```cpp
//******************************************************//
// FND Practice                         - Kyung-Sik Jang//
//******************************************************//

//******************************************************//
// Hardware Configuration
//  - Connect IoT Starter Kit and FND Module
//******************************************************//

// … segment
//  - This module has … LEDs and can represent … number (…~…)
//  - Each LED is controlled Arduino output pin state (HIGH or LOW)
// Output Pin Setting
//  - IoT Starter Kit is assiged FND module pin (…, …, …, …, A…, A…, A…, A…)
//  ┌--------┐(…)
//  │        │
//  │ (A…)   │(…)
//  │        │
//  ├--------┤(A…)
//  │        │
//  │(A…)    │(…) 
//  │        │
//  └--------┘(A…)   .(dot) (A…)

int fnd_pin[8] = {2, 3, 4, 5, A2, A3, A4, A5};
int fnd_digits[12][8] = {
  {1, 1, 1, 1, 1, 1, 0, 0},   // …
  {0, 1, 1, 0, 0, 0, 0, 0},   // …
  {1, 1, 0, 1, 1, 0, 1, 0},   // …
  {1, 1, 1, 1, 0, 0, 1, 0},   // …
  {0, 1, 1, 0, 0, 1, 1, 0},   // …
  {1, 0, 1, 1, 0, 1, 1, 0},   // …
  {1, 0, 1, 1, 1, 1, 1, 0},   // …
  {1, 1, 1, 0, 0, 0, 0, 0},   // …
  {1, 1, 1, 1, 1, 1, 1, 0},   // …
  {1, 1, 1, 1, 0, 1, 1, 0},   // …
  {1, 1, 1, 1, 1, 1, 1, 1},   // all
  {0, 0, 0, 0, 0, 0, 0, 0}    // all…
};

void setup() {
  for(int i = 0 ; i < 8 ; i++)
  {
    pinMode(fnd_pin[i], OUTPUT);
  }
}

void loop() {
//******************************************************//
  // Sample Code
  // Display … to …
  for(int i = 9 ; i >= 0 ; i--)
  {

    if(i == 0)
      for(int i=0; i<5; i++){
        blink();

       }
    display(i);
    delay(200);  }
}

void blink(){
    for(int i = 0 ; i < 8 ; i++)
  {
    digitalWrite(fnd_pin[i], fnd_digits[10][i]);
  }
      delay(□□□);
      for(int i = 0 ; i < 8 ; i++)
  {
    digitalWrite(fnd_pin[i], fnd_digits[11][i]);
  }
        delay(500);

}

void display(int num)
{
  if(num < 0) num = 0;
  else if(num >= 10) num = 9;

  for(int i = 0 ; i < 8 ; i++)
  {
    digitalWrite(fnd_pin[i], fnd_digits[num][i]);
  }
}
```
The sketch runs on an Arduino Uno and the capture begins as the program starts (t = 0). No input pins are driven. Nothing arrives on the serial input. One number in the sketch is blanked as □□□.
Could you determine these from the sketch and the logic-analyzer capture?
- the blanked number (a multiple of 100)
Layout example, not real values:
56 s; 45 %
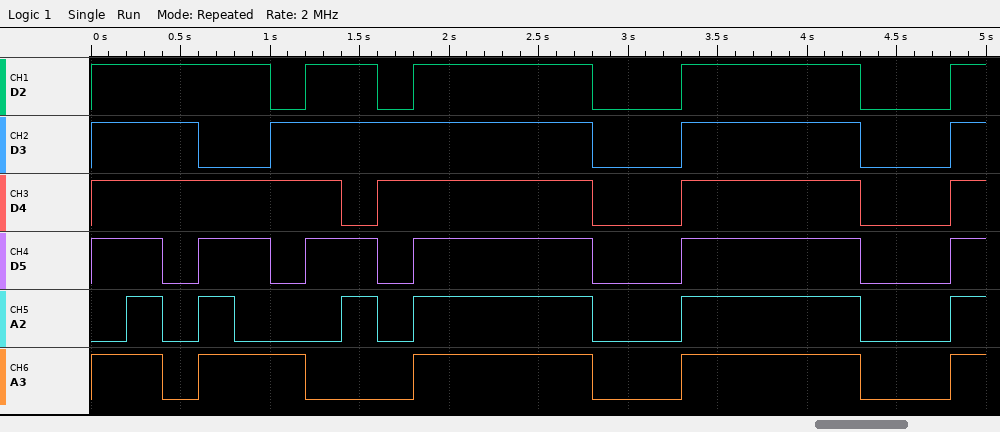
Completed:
1000
